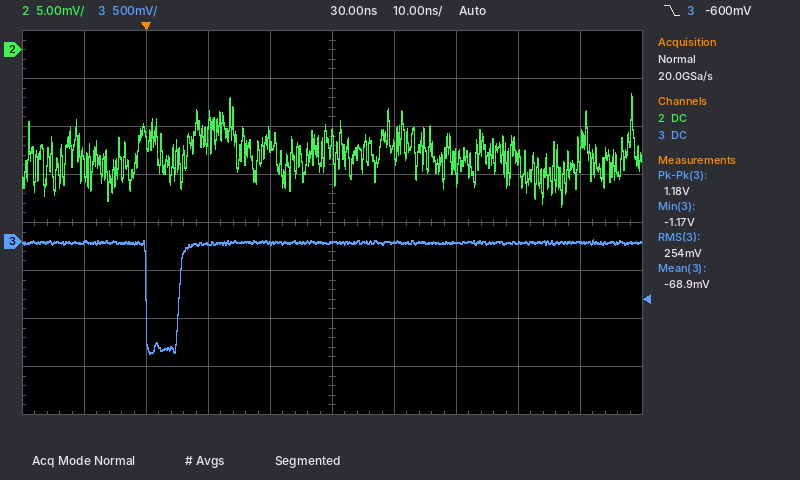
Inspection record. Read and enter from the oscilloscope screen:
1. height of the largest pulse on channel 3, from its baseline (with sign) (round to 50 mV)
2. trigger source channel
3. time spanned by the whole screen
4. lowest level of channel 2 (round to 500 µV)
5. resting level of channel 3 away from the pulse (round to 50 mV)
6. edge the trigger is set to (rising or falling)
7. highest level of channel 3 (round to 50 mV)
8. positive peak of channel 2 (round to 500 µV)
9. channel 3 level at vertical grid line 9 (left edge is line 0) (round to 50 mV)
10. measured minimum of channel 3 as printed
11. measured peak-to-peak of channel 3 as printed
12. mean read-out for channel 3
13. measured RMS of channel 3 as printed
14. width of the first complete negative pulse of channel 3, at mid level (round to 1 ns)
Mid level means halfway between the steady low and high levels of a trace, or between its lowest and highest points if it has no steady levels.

-1.15 V
channel 3
100 ns
-16.5 mV
0 mV
falling
0 mV
-4.5 mV
0 mV
-1.17 V
1.18 V
-68.9 mV
254 mV
5 ns
